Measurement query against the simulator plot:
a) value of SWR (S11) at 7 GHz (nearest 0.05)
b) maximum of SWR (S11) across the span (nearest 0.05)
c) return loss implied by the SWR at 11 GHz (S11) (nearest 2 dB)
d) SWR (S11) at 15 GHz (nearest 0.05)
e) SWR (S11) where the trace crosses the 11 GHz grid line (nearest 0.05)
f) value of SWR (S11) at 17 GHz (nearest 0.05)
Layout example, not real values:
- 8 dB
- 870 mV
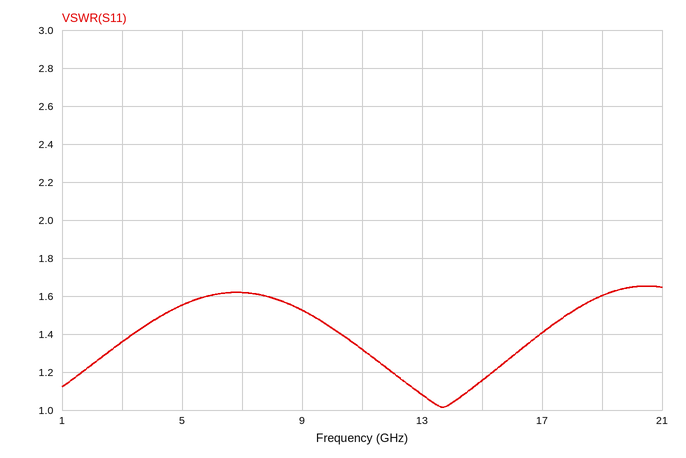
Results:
- 1.60
- 1.65
- 18 dB
- 1.15
- 1.30
- 1.40
